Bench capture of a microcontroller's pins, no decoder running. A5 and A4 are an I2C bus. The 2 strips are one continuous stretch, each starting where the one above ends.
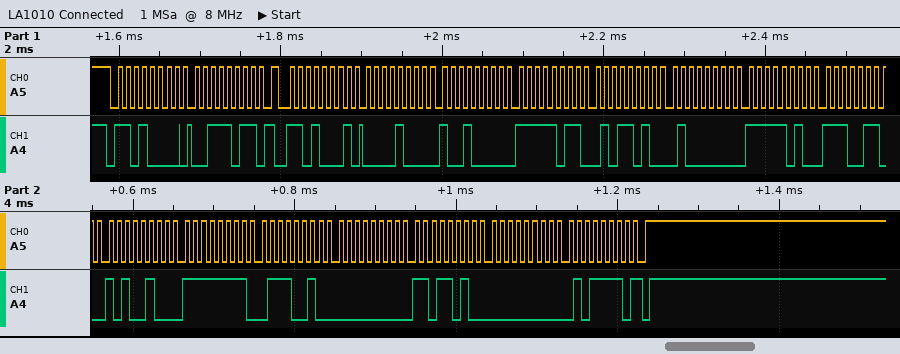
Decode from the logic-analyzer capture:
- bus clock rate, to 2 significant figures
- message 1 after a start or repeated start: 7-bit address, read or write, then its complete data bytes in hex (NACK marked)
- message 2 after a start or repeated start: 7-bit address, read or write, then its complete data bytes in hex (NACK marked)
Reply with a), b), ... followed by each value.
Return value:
a) 100 kHz
b) 0x68 write: 3B
c) 0x68 read: 08 90 FB 5A 40 FA E6 A4 FF 72 00 DA 00 5E NACK
